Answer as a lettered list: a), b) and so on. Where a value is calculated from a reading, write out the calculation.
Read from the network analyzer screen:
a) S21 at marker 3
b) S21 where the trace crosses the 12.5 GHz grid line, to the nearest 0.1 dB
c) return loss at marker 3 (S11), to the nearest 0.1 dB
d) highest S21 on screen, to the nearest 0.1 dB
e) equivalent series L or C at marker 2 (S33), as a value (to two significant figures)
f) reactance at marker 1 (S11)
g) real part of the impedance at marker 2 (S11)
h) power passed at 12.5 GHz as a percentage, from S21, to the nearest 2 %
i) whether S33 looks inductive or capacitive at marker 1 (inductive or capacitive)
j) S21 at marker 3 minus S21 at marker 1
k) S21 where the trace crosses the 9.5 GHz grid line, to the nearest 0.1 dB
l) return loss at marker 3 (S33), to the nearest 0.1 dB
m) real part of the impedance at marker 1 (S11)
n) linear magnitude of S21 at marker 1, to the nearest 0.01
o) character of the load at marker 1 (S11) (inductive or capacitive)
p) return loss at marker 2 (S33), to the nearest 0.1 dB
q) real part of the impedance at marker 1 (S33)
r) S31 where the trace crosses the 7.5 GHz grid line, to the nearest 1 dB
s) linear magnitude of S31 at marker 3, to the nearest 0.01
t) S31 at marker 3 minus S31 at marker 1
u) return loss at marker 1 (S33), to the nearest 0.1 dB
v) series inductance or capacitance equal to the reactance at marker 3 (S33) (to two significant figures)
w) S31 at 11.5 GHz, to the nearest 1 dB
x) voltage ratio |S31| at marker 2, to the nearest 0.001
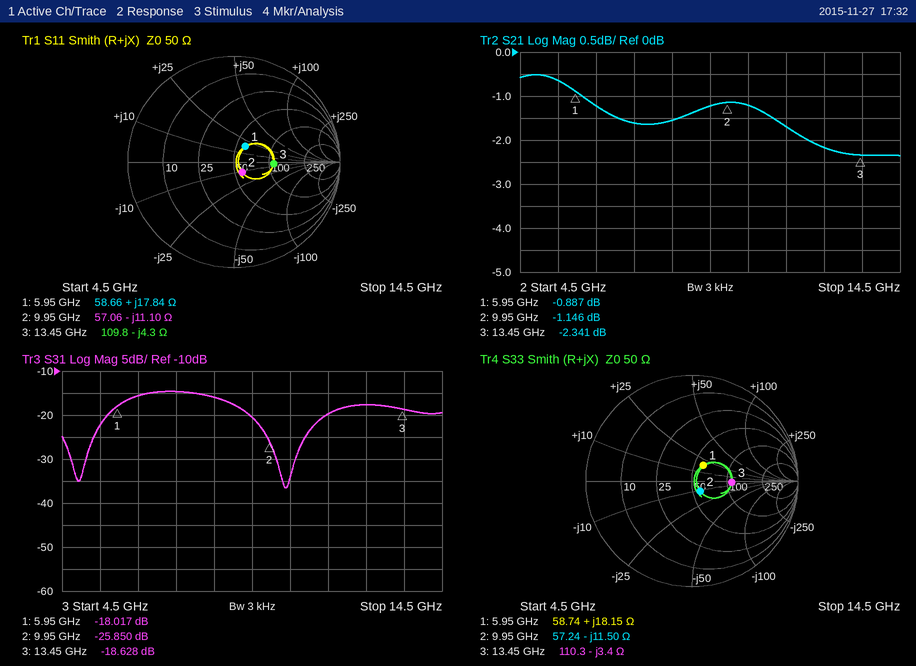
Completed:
a) -2.341 dB
b) -2.2 dB
c) 8.5 dB
d) -0.5 dB
e) C = 1/(2π × 9.95 GHz × 11.5 Ω) ≈ 1.4 pF
f) +17.84 Ω
g) 57.06 Ω
h) 10^(-2.2/10) ≈ 60 %
i) inductive
j) -2.341 − (-0.887) = -1.454 dB
k) -1.2 dB
l) 8.5 dB
m) 58.66 Ω
n) 10^(-0.887/20) ≈ 0.90
o) inductive
p) 18.0 dB
q) 58.74 Ω
r) -15 dB
s) 10^(-18.628/20) ≈ 0.12
t) -18.628 − (-18.017) = -0.611 dB
u) 14.8 dB
v) C = 1/(2π × 13.45 GHz × 3.4 Ω) ≈ 3.5 pF
w) -20 dB
x) 10^(-25.85/20) ≈ 0.051
